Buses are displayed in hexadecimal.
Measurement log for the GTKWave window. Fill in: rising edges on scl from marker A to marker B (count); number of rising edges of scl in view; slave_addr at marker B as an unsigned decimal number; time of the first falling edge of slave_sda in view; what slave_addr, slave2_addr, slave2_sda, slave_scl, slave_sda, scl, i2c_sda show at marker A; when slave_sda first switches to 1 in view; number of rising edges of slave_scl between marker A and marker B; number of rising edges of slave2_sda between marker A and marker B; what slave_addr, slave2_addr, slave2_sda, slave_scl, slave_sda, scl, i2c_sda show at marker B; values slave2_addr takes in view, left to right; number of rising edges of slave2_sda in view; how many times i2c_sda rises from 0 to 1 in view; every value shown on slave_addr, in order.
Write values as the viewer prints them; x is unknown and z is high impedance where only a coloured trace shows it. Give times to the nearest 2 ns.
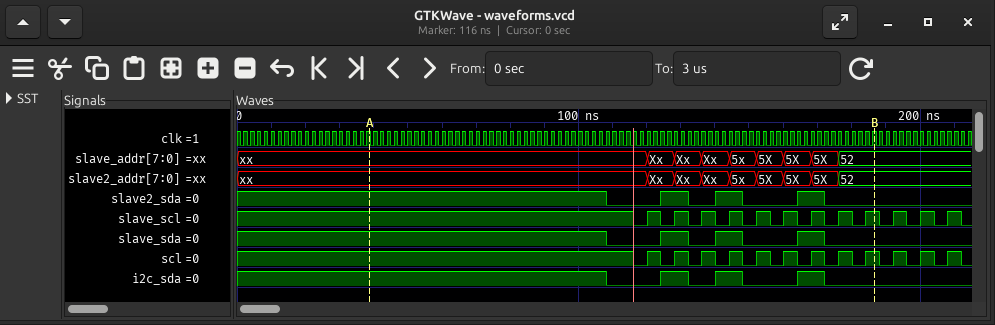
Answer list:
9
12
82
108 ns
slave_addr=xx, slave2_addr=xx, slave2_sda=1, slave_scl=1, slave_sda=1, scl=1, i2c_sda=1
124 ns
9
3
slave_addr=52, slave2_addr=52, slave2_sda=0, slave_scl=1, slave_sda=0, scl=1, i2c_sda=0
xx, Xx, Xx, Xx, 5x, 5X, 5X, 5X, 52
3
3
xx, Xx, Xx, Xx, 5x, 5X, 5X, 5X, 52
